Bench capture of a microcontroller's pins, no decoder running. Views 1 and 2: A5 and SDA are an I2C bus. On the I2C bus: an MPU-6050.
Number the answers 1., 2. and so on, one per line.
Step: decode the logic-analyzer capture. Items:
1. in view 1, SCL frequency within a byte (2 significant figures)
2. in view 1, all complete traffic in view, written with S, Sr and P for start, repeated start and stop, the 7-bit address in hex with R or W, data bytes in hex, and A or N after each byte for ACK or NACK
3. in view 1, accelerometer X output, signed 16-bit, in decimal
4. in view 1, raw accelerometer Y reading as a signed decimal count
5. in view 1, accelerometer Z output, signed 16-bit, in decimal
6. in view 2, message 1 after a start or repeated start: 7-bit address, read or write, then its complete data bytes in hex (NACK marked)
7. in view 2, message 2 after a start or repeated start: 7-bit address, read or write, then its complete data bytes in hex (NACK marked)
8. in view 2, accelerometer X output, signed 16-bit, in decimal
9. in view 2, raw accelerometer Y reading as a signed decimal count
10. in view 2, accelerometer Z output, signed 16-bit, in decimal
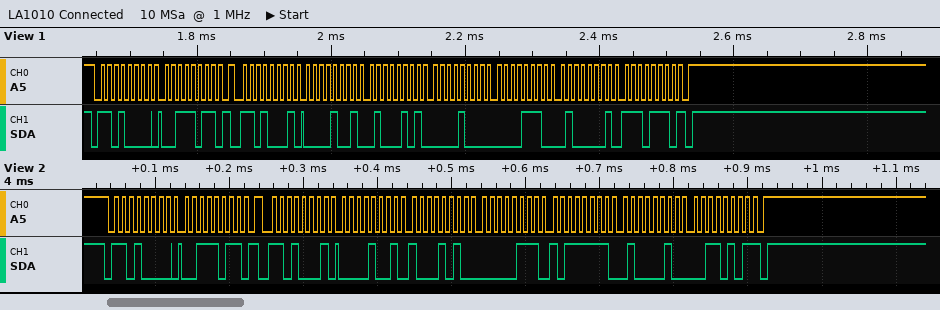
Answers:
1. 100 kHz
2. S 68W A 3B A Sr 68R A 09 A 45 A 08 A 0E A 41 A EE N P
3. 2373
4. 2062
5. 16878
6. 0x68 write: 3B
7. 0x68 read: 09 8A 07 BF 42 35 NACK
8. 2442
9. 1983
10. 16949
